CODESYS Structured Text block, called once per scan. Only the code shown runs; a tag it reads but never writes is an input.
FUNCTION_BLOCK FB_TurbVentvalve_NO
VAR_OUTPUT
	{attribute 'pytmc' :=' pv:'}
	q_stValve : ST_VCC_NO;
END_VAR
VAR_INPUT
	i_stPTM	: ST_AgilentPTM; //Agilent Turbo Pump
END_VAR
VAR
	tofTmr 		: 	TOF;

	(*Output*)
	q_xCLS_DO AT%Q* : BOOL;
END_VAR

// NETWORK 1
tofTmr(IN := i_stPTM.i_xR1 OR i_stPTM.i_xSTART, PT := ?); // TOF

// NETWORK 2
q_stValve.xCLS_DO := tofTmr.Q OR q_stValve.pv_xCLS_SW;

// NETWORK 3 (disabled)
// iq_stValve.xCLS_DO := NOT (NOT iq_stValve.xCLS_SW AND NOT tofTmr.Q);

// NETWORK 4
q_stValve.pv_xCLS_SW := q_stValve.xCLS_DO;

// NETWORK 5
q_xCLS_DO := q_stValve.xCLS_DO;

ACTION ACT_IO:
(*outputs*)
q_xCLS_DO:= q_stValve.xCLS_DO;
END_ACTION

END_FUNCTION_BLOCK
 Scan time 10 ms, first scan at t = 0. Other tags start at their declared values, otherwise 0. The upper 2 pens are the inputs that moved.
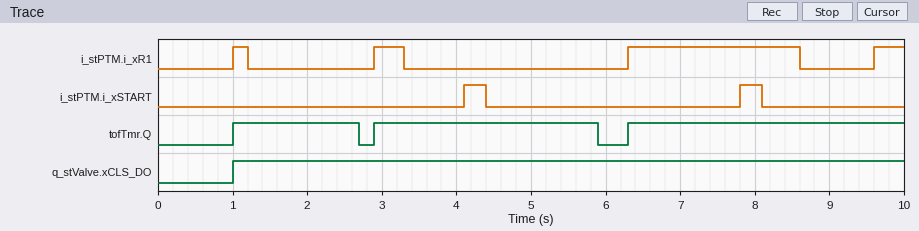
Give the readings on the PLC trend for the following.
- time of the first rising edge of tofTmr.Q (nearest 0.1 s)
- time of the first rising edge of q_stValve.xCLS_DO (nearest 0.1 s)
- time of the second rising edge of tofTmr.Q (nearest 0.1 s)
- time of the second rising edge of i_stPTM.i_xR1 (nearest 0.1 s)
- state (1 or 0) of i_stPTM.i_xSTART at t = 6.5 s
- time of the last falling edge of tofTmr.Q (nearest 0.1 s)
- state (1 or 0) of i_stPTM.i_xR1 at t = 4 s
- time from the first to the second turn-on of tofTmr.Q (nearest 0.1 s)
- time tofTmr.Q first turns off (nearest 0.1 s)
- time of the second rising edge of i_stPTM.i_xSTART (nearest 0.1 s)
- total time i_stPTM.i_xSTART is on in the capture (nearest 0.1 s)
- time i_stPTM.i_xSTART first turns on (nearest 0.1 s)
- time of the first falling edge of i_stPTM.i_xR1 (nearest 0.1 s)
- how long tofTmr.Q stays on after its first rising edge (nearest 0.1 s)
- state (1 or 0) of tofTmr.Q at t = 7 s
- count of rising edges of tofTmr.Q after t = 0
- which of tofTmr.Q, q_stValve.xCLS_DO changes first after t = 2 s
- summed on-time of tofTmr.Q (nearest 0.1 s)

1.0 s
1.0 s
2.9 s
2.9 s
0
5.9 s
0
1.9 s
2.7 s
7.8 s
0.6 s
4.1 s
1.2 s
1.7 s
1
3
tofTmr.Q
8.4 s
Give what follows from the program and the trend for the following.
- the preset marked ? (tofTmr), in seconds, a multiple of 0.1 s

1.5 s
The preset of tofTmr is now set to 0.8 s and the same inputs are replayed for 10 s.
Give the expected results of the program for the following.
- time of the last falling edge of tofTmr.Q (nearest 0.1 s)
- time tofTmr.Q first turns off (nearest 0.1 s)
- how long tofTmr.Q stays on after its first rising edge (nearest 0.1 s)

9.4 s
2.0 s
1.0 s
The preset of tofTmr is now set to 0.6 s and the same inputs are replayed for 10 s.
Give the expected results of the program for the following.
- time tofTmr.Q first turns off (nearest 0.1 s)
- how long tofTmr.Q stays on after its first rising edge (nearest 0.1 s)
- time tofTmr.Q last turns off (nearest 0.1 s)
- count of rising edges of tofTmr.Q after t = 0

1.8 s
0.8 s
9.2 s
5
